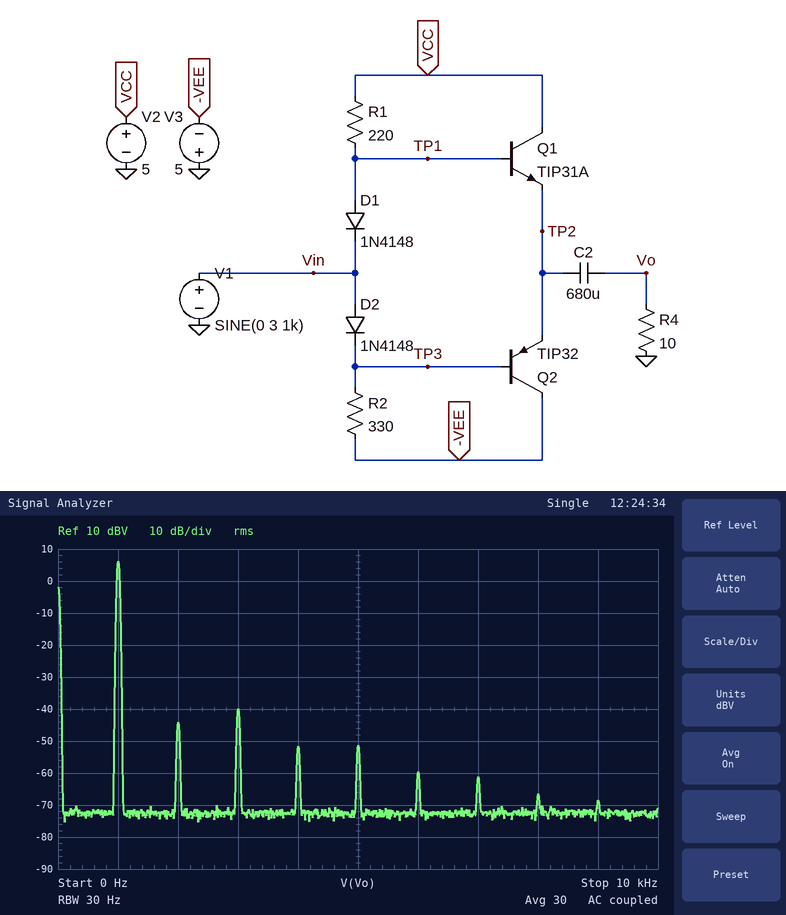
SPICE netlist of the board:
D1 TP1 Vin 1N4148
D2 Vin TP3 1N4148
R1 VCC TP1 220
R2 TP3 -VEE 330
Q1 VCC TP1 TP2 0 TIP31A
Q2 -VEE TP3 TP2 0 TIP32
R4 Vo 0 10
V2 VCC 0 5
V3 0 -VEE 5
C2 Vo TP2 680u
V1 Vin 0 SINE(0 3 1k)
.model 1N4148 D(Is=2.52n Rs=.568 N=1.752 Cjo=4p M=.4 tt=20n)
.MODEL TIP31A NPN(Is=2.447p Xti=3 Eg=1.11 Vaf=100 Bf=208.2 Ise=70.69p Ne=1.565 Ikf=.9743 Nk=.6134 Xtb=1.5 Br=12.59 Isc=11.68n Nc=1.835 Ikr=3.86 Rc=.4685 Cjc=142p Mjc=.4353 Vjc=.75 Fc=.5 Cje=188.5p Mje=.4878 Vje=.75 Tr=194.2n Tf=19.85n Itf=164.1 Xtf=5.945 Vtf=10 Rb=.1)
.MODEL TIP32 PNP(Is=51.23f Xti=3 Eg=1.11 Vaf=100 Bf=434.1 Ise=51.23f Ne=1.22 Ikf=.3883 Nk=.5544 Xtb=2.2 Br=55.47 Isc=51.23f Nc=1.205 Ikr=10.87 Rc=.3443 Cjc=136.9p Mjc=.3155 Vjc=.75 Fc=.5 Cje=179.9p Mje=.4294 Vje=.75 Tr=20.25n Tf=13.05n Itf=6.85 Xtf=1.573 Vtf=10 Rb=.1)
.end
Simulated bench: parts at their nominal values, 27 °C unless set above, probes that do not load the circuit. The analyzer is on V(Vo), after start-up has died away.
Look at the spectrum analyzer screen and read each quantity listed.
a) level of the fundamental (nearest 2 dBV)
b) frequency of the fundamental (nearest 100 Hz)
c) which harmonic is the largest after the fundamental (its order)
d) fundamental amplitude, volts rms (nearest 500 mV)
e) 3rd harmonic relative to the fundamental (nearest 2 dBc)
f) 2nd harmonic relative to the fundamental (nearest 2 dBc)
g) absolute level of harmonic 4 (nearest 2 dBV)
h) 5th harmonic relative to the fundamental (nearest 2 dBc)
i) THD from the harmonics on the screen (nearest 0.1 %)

6 dBV
1.0 kHz
3
2.0 V
-46 dBc
-50 dBc
-52 dBV
-58 dBc
0.6 %
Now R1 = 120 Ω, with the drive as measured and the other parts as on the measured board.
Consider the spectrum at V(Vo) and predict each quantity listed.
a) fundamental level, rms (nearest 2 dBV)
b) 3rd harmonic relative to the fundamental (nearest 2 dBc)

6 dBV
-48 dBc
